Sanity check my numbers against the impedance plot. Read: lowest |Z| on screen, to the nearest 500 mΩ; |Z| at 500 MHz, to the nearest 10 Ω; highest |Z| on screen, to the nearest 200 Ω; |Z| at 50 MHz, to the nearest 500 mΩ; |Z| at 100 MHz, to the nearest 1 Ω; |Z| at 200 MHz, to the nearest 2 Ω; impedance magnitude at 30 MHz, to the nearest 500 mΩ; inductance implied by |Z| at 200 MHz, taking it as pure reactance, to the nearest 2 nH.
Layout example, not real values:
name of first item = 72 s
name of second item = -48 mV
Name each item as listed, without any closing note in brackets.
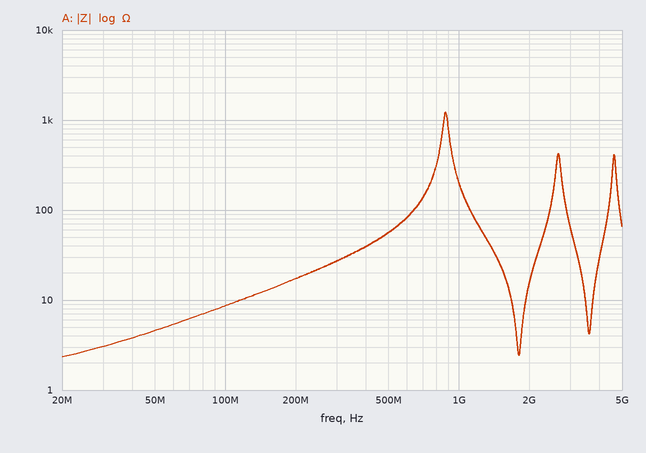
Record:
lowest |Z| on screen, to the nearest 500 mΩ = 2.5 Ω
|Z| at 500 MHz, to the nearest 10 Ω = 60 Ω
highest |Z| on screen, to the nearest 200 Ω = 1.2 kΩ
|Z| at 50 MHz, to the nearest 500 mΩ = 4.5 Ω
|Z| at 100 MHz, to the nearest 1 Ω = 9 Ω
|Z| at 200 MHz, to the nearest 2 Ω = 18 Ω
impedance magnitude at 30 MHz, to the nearest 500 mΩ = 3.0 Ω
inductance implied by |Z| at 200 MHz, taking it as pure reactance, to the nearest 2 nH = 14 nH
